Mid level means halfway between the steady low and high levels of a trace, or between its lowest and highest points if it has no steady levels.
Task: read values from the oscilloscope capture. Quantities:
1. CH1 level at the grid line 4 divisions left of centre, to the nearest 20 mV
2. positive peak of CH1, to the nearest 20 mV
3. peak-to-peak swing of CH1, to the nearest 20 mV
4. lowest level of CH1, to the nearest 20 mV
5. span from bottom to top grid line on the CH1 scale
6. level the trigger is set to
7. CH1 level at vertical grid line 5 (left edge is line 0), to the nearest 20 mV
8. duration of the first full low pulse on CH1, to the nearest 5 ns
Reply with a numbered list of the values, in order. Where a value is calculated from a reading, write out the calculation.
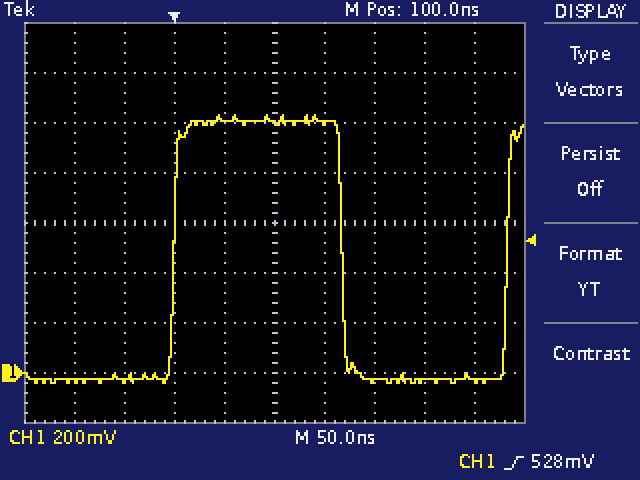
1. -40 mV
2. 1.04 V
3. 1.04 V − (-40 mV) = 1.08 V
4. -40 mV
5. 1.6 V
6. 528 mV
7. 1.00 V
8. 165 ns
